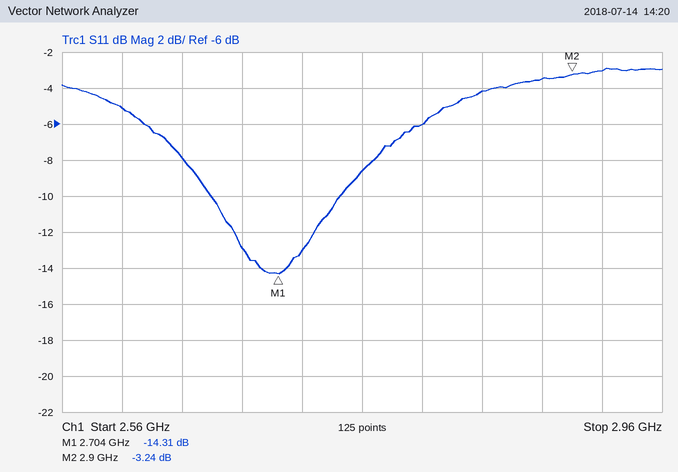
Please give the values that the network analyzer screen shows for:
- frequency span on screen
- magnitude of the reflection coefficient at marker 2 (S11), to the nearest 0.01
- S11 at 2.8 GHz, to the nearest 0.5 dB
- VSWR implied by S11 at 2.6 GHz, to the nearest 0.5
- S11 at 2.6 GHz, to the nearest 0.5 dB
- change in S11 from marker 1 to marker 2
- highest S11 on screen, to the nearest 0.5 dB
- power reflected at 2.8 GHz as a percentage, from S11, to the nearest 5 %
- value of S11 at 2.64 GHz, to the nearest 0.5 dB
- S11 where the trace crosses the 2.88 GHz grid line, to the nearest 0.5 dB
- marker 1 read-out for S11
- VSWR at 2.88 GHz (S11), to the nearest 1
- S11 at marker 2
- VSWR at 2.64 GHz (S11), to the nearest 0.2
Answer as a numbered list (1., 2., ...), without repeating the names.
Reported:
1. 400 MHz
2. 0.69
3. -6.0 dB
4. 3.5
5. -5.0 dB
6. 11.07 dB
7. -3.0 dB
8. 25 %
9. -8.0 dB
10. -3.5 dB
11. -14.31 dB
12. 5
13. -3.24 dB
14. 2.4
